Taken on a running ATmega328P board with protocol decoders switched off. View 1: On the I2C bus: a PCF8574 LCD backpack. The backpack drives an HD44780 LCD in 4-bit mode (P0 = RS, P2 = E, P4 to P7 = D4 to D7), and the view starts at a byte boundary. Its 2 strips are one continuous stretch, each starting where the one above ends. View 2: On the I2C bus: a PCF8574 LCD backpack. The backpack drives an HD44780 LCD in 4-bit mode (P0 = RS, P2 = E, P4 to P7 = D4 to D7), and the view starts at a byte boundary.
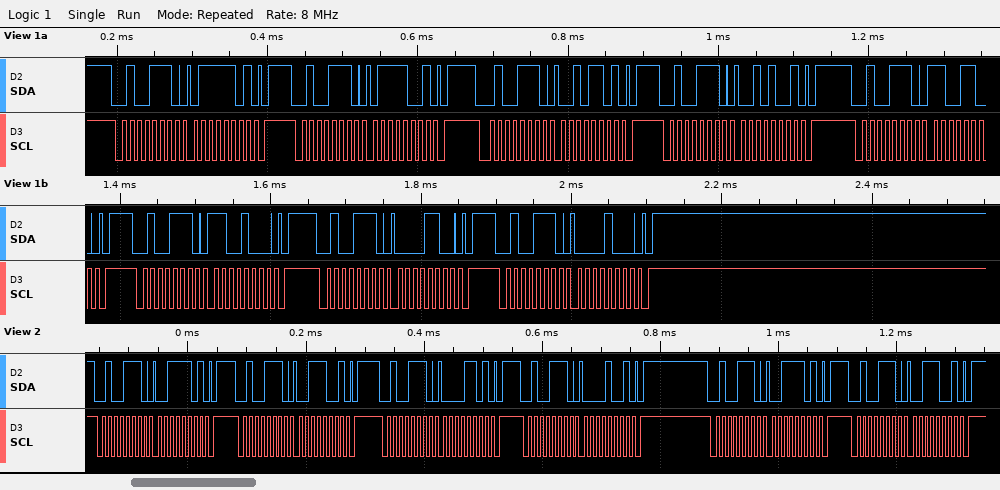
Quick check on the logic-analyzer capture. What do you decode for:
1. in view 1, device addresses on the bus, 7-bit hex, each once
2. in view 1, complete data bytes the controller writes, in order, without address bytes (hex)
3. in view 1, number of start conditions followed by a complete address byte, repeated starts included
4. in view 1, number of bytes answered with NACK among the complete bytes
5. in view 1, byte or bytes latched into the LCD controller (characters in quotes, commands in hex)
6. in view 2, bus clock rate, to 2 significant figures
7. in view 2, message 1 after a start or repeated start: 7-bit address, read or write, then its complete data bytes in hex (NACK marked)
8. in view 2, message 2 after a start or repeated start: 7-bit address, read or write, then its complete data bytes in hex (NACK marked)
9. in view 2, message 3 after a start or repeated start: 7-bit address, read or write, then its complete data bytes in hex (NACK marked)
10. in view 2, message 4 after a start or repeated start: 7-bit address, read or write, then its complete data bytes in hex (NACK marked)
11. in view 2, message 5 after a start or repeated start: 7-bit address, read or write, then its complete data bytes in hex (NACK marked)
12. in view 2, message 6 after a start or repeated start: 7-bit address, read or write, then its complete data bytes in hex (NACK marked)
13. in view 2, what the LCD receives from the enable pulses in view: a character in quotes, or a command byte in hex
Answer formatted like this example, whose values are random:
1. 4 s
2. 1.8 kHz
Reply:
1. 0x27
2. 7D 79 2D 29 CC C8 0C 08
3. 8
4. 0
5. 'r' 0xC0
6. 100 kHz
7. 0x27 write: 3D
8. 0x27 write: 39
9. 0x27 write: 0D
10. 0x27 write: 09
11. 0x27 write: 3D
12. 0x27 write: 39
13. '0'
